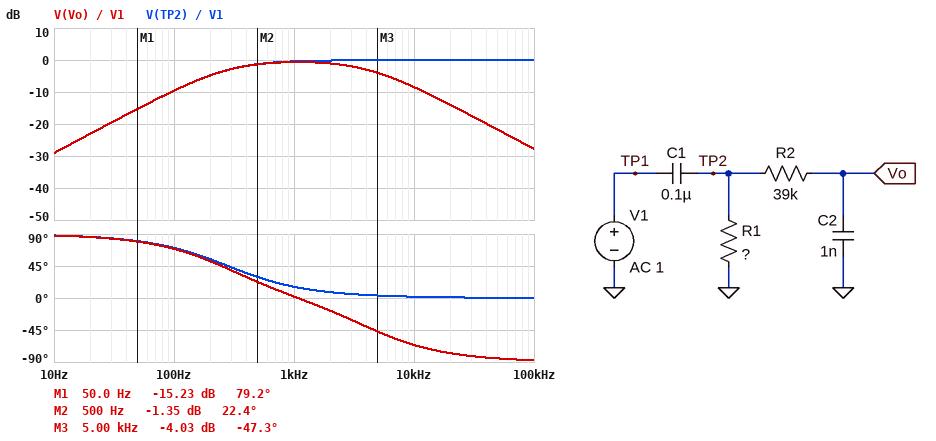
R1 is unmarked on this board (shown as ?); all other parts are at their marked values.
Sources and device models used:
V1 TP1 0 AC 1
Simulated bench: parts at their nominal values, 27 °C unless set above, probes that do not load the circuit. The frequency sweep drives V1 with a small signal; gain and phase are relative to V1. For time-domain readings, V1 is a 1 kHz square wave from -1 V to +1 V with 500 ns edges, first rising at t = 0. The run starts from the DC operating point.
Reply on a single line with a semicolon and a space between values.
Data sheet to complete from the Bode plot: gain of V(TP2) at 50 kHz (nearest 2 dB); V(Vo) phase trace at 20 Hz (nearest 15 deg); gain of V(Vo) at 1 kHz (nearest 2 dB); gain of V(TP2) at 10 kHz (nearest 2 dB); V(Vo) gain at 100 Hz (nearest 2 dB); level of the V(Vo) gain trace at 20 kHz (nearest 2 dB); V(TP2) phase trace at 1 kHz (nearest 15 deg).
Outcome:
0 dB; 90 deg; 0 dB; 0 dB; -10 dB; -14 dB; 15 deg
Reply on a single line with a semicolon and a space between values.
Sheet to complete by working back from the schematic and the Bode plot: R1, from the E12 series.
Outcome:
5.6 kΩ
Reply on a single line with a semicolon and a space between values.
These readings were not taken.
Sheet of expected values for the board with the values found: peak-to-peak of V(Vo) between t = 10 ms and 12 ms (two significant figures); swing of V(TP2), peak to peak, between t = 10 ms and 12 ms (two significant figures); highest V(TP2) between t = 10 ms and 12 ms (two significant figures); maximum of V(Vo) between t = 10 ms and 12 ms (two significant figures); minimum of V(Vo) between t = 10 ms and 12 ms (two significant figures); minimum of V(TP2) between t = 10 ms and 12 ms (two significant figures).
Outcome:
2.2 V; 2.8 V; 1.4 V; 1.1 V; -1.1 V; -1.4 V
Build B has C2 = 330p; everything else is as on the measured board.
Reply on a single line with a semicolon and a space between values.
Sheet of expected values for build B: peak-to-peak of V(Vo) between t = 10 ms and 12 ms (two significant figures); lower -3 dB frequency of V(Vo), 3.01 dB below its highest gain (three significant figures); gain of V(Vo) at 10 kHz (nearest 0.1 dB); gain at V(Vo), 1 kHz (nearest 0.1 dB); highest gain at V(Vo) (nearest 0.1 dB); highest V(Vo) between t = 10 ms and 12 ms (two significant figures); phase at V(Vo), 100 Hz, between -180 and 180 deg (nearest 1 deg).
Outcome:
2.6 V; 271 Hz; -2.2 dB; -0.4 dB; -0.2 dB; 1.3 V; 70 deg
